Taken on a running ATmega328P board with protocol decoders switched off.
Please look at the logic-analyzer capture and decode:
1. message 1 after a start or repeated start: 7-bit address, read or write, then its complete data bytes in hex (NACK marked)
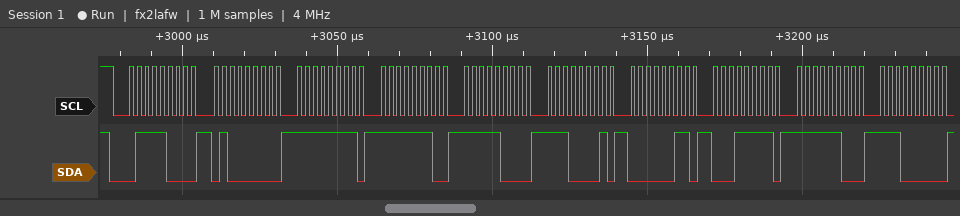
0x3C write: 40 FF FE F8 E1 03 1F FC E0
